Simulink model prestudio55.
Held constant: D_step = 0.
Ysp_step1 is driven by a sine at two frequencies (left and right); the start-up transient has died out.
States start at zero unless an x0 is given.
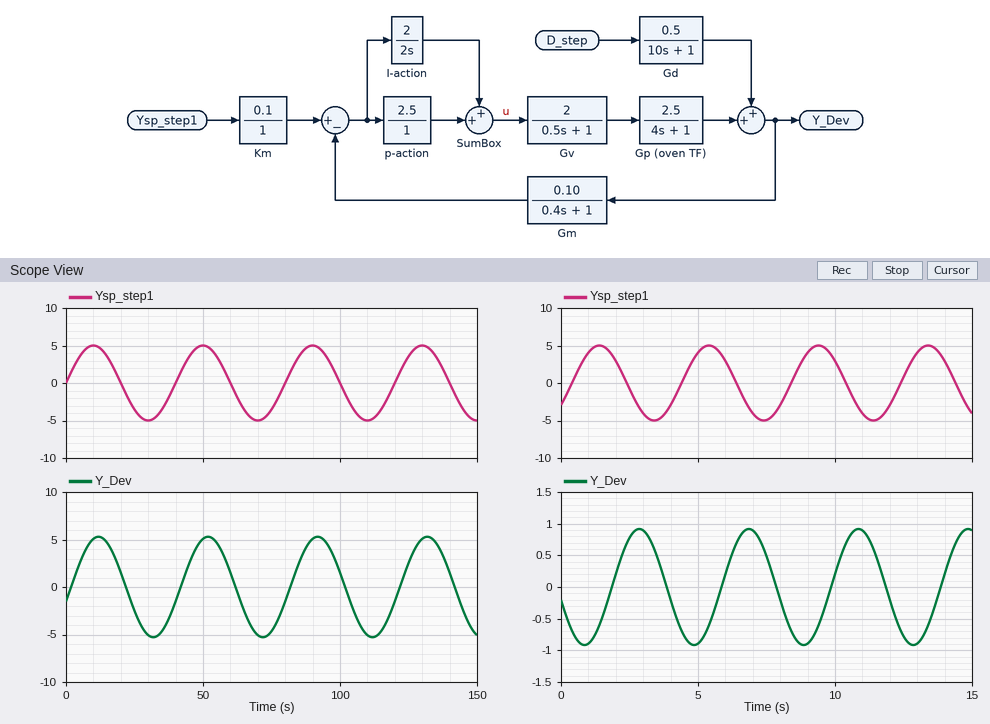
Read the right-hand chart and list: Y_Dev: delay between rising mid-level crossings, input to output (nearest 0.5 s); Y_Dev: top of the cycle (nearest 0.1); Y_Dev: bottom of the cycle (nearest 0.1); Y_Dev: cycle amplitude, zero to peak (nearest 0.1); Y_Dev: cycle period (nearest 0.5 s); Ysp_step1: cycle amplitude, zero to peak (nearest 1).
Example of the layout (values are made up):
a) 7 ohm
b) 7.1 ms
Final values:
a) 1.5 s
b) 0.9
c) -0.9
d) 0.9
e) 4.0 s
f) 5
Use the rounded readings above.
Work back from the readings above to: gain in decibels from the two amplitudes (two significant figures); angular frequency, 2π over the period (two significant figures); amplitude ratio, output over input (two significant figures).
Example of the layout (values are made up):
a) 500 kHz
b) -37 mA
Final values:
a) -15 dB
b) 1.6 rad/s
c) 0.18
